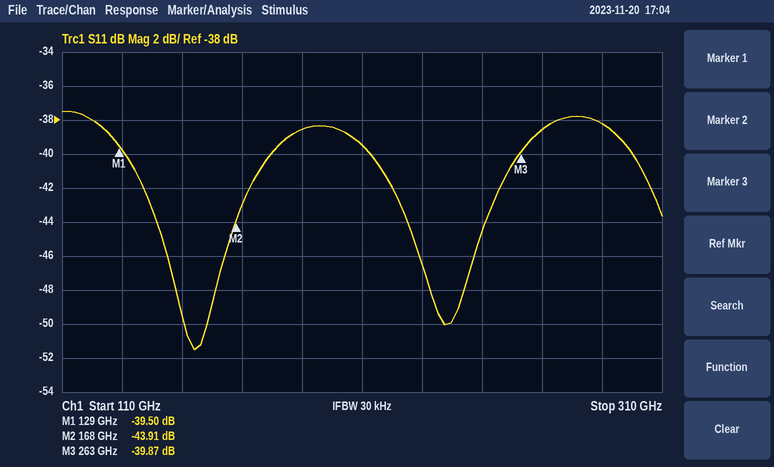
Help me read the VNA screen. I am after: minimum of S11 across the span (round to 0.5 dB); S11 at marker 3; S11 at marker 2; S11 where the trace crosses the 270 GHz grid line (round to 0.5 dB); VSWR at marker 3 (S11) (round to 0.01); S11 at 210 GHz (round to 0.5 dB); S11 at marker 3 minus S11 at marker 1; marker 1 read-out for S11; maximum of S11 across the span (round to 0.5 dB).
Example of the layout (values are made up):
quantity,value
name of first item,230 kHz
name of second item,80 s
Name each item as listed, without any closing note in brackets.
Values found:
quantity,value
minimum of S11 across the span,-51.5 dB
S11 at marker 3,-39.87 dB
S11 at marker 2,-43.91 dB
S11 where the trace crosses the 270 GHz grid line,-38.5 dB
VSWR at marker 3 (S11),1.02
S11 at 210 GHz,-39.5 dB
S11 at marker 3 minus S11 at marker 1,-0.37 dB
marker 1 read-out for S11,-39.50 dB
maximum of S11 across the span,-37.5 dB
